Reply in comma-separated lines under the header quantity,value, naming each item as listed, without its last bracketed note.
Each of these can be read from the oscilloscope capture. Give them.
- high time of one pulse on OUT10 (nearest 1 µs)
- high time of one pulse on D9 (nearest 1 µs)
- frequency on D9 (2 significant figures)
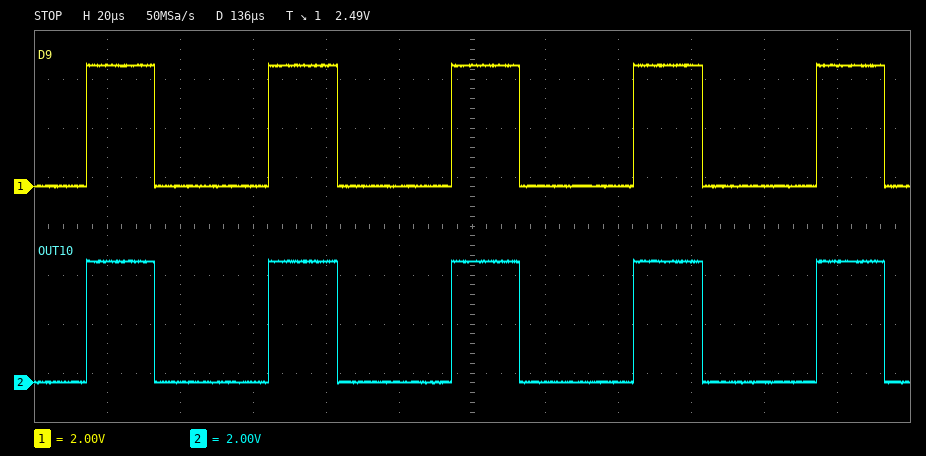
quantity,value
high time of one pulse on OUT10,19 µs
high time of one pulse on D9,19 µs
frequency on D9,20 kHz
